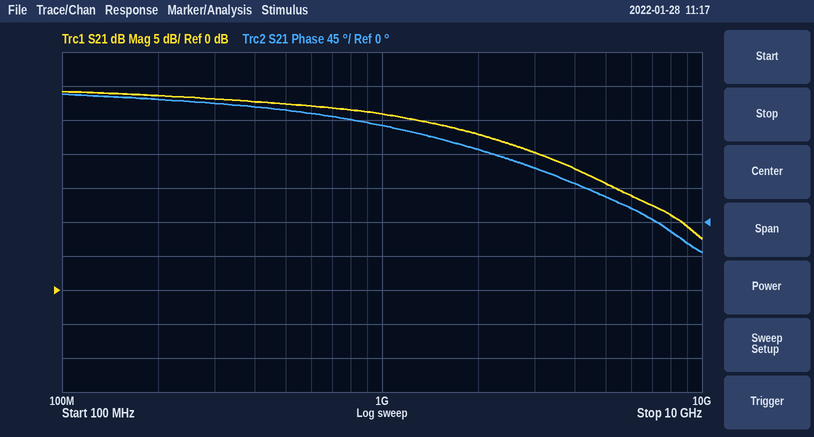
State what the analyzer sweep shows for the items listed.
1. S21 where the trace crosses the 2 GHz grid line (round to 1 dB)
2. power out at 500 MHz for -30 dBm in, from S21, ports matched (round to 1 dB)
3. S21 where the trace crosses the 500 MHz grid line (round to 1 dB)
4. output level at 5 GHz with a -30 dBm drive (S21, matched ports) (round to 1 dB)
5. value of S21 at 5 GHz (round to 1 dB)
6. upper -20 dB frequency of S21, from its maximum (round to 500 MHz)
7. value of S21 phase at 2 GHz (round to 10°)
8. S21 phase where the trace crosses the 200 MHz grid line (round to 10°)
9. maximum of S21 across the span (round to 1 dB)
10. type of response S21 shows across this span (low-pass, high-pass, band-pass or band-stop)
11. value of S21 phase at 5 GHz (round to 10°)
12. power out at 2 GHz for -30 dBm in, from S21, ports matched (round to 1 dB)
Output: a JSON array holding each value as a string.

["23 dB", "-3 dBm", "27 dB", "-14 dBm", "16 dB", "9.0 GHz", "100°", "160°", "29 dB", "low-pass", "30°", "-7 dBm"]
